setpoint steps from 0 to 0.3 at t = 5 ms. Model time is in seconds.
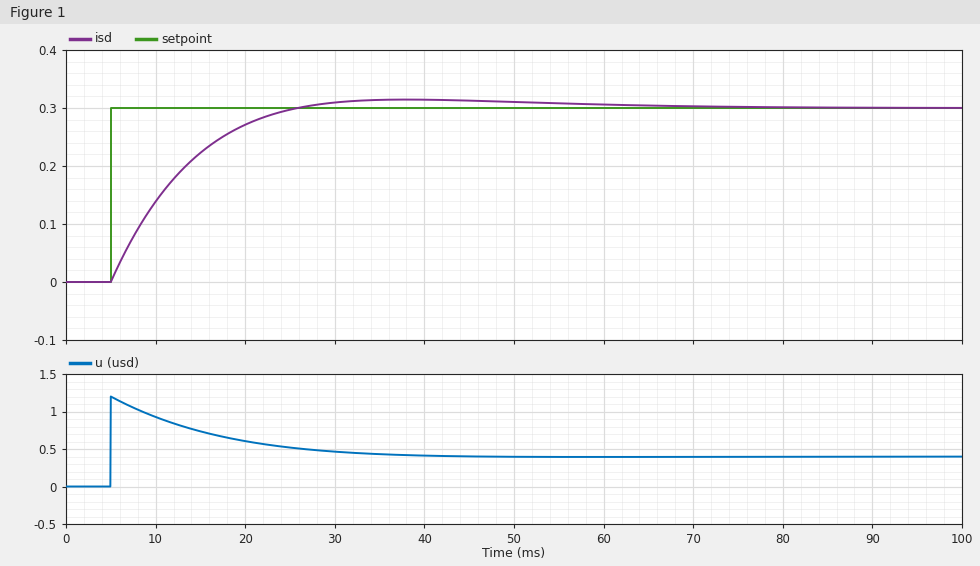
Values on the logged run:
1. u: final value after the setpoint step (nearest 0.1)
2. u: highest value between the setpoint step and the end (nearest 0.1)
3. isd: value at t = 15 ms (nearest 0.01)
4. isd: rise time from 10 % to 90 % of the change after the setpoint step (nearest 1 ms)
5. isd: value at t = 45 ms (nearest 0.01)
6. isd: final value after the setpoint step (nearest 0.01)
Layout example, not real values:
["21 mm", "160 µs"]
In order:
["0.4", "1.2", "0.22", "14 ms", "0.31", "0.30"]
